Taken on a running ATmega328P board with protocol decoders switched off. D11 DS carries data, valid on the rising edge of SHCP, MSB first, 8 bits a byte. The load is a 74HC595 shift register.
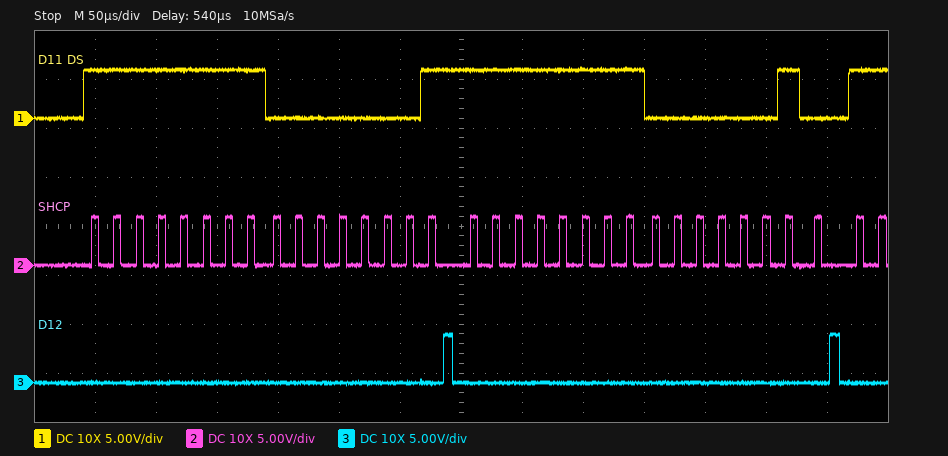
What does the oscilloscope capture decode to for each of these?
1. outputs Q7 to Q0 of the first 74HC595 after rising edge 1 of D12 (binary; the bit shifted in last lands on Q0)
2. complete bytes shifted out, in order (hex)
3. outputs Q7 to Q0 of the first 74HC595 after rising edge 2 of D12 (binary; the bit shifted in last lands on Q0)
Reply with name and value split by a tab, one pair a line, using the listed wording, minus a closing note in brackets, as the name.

outputs Q7 to Q0 of the first 74HC595 after rising edge 1 of D12	00000001
complete bytes shifted out, in order	FF 01 FF 02
outputs Q7 to Q0 of the first 74HC595 after rising edge 2 of D12	00000010
